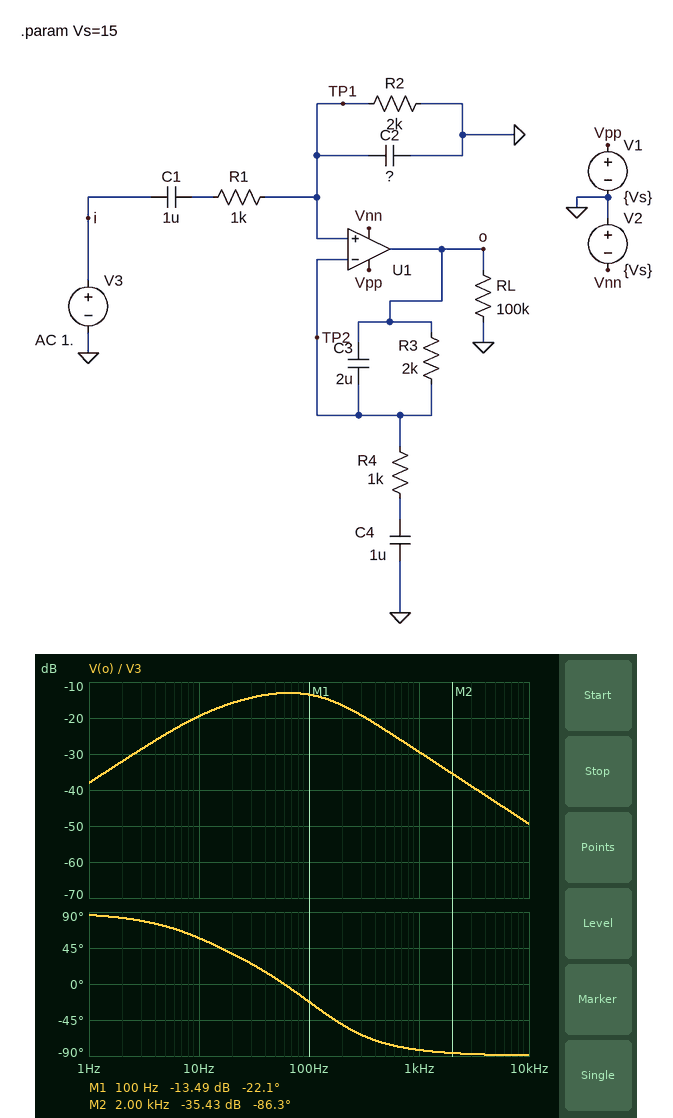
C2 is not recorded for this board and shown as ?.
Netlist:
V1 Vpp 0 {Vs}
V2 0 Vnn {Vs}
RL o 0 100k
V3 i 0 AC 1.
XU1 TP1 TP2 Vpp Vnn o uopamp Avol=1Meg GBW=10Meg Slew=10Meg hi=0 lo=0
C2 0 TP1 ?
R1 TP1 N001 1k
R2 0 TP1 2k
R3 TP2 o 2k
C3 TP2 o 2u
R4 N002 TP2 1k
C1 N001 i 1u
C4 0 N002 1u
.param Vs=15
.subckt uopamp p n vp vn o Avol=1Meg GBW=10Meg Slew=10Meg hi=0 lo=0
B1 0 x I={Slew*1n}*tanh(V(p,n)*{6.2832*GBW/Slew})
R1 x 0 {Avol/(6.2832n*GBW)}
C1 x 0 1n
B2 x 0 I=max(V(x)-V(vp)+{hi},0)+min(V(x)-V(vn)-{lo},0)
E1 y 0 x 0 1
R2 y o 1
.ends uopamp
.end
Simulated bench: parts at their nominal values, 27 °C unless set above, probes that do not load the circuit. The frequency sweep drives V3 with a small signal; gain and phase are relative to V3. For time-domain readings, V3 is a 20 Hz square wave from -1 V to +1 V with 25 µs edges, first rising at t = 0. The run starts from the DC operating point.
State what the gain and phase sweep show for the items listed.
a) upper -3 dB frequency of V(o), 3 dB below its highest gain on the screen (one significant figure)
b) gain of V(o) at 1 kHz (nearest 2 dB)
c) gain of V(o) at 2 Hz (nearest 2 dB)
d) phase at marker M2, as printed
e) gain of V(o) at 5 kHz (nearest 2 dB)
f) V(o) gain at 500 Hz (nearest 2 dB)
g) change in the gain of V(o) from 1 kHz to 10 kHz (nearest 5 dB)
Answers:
200 Hz
-30 dB
-32 dB
-86.3 deg
-44 dB
-24 dB
-20 dB
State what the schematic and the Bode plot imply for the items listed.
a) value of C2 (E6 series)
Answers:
4.7 µF
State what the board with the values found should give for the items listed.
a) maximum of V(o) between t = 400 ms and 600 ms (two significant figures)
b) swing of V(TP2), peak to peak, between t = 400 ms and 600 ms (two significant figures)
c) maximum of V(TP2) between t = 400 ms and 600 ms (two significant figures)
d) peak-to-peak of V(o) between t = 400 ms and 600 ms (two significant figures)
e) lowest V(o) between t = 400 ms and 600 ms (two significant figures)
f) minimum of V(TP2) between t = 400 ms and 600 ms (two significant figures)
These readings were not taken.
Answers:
350 mV
500 mV
250 mV
690 mV
-350 mV
-250 mV
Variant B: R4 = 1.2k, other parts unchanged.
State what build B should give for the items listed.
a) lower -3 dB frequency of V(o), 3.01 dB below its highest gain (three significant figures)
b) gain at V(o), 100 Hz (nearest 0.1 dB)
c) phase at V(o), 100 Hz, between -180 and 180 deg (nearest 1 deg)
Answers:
18.8 Hz
-13.7 dB
-23 deg
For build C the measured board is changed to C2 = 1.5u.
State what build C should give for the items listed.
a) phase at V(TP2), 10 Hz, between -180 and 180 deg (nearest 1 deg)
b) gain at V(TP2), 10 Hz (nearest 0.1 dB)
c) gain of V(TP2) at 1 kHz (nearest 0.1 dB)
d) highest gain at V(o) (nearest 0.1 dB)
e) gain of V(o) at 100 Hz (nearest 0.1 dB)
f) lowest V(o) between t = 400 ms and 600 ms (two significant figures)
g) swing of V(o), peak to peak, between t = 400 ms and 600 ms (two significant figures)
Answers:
69 deg
-18.5 dB
-19.8 dB
-6.6 dB
-6.7 dB
-730 mV
1.5 V
